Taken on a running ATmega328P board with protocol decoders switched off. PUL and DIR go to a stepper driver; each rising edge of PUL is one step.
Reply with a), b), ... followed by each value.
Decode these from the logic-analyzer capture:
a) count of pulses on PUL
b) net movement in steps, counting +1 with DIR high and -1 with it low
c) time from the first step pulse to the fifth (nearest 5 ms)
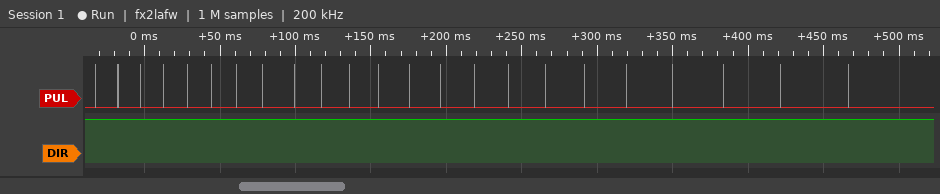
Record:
a) 23
b) +23
c) 60 ms
